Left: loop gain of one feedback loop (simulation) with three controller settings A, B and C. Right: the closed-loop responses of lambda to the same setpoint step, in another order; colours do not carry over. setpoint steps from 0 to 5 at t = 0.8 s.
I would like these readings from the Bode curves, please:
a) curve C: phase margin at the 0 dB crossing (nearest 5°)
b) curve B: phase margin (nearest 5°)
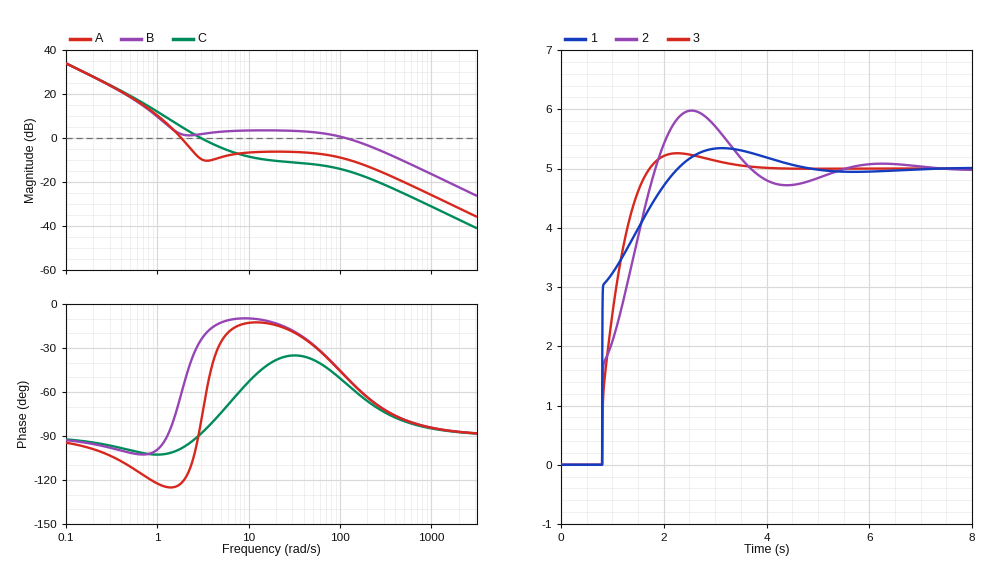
90°
130°
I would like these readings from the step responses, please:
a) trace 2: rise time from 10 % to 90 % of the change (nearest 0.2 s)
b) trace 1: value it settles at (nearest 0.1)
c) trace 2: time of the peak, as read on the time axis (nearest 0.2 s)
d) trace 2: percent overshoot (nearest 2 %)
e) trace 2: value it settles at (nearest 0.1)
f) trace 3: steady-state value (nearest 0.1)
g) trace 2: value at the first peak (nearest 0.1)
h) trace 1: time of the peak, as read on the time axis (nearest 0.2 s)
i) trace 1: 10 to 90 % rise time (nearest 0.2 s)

0.8 s
5.0
2.6 s
20 %
5.0
5.0
6.0
3.2 s
1.0 s
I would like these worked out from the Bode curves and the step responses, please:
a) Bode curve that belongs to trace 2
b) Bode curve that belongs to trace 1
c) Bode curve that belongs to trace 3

A
B
C
